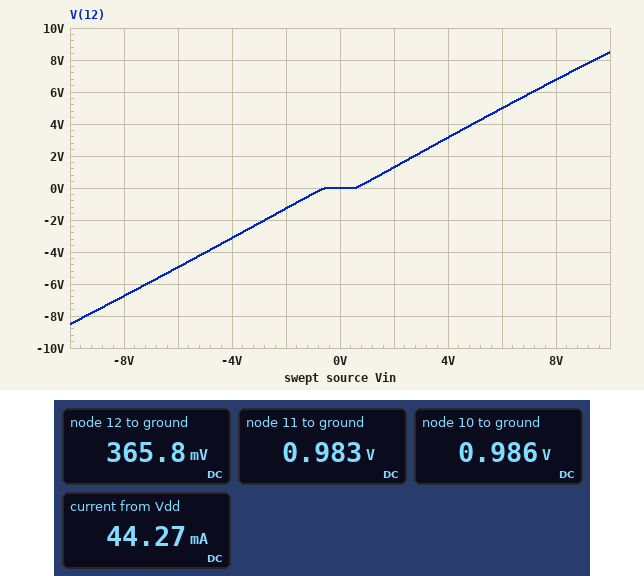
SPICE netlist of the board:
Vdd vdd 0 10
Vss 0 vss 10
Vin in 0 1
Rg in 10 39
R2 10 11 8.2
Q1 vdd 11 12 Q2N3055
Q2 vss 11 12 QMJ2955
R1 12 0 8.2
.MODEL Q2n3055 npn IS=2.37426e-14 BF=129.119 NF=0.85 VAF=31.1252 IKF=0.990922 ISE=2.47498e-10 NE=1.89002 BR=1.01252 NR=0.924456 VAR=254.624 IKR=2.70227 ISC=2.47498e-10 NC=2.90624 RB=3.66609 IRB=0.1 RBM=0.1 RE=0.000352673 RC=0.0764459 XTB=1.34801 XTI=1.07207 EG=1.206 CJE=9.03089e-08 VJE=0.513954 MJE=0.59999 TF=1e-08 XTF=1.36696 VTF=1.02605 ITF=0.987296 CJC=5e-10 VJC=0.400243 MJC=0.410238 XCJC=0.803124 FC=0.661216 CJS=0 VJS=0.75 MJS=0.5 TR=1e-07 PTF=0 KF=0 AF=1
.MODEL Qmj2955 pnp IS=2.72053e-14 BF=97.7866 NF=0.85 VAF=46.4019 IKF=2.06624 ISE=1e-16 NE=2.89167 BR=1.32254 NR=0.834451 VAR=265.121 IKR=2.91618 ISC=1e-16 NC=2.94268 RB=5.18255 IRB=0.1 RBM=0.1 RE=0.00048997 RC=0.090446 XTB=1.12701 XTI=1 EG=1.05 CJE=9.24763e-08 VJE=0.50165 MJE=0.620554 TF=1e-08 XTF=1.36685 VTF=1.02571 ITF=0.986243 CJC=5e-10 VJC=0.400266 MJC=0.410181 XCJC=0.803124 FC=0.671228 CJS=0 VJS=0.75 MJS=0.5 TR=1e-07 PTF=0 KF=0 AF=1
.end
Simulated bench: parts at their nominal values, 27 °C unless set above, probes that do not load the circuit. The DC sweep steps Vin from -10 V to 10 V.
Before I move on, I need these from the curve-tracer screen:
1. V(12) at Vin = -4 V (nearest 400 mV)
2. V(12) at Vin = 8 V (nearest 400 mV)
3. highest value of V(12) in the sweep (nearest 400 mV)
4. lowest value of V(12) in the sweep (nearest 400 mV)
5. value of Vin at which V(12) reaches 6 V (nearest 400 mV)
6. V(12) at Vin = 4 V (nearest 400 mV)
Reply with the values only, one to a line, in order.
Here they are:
-3.2 V
6.8 V
8.4 V
-8.4 V
7.2 V
3.2 V
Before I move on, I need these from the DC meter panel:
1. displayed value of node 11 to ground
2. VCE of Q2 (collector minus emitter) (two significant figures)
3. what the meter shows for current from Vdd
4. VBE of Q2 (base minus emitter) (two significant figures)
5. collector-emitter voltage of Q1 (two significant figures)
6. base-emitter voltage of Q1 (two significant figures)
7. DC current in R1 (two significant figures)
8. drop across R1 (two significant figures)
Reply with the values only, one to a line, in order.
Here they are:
0.983 V
-10 V
44.27 mA
620 mV
9.6 V
620 mV
45 mA
370 mV
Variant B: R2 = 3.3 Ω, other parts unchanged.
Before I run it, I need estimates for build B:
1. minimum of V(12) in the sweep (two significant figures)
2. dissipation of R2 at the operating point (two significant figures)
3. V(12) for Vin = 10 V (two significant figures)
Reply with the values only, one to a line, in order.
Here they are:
-8.6 V
410 nW
8.6 V
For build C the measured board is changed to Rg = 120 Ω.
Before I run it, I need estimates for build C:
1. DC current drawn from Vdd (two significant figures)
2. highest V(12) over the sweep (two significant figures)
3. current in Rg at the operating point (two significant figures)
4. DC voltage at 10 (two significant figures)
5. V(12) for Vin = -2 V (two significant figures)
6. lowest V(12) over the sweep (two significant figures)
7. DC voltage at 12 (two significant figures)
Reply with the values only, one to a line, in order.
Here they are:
41 mA
7.6 V
330 µA
960 mV
-1.2 V
-7.6 V
340 mV
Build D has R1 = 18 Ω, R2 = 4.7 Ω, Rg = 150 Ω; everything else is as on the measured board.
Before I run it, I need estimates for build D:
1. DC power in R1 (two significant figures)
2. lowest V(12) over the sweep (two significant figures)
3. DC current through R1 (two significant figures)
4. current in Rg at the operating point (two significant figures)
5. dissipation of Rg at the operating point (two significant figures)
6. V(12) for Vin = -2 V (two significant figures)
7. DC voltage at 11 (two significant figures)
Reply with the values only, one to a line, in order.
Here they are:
7.7 mW
-8.4 V
21 mA
180 µA
4.7 µW
-1.3 V
970 mV
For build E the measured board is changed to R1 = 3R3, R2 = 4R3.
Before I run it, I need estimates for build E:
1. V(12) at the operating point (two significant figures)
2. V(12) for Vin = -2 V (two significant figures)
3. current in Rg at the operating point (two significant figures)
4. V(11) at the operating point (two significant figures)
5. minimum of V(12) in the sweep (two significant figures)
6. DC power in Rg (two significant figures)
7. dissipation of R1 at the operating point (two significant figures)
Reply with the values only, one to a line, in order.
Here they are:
330 mV
-1.2 V
750 µA
970 mV
-7.3 V
22 µW
33 mW
